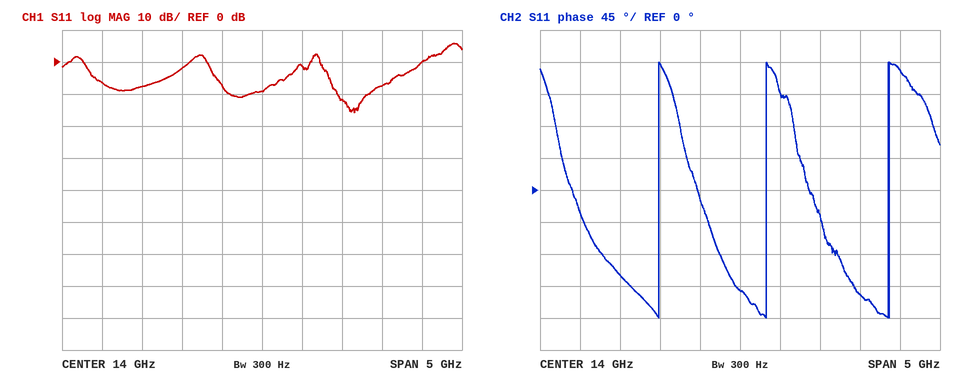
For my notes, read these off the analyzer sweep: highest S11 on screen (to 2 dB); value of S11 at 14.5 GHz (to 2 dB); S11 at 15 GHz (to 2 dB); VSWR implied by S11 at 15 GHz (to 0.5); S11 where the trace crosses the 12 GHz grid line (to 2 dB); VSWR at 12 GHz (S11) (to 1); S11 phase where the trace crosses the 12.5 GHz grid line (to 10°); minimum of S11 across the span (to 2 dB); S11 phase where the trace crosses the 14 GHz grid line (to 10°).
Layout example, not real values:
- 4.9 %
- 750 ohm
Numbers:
- 6 dB
- -2 dB
- -12 dB
- 1.5
- -6 dB
- 3
- -120°
- -16 dB
- -140°
